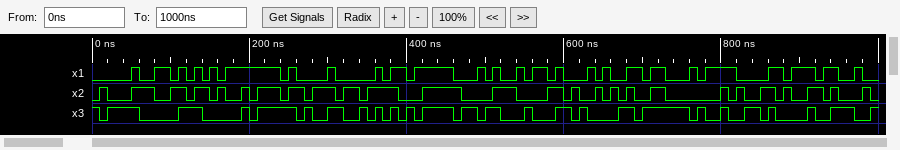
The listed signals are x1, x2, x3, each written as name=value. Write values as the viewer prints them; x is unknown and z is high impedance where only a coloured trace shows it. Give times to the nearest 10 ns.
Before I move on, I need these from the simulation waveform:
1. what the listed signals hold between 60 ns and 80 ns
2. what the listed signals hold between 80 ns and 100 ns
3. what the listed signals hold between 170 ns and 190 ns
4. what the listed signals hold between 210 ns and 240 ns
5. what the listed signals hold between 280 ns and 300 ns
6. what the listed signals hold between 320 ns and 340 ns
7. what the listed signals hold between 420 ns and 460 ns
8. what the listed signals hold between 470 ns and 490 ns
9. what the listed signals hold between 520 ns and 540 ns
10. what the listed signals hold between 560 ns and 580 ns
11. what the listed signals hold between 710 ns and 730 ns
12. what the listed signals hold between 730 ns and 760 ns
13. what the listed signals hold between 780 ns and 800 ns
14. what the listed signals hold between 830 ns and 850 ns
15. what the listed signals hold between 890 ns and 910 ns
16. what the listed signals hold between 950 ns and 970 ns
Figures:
x1=0, x2=1, x3=0
x1=1, x2=0, x3=0
x1=1, x2=0, x3=0
x1=1, x2=1, x3=1
x1=0, x2=1, x3=0
x1=0, x2=1, x3=0
x1=1, x2=1, x3=1
x1=0, x2=0, x3=1
x1=0, x2=1, x3=0
x1=1, x2=0, x3=0
x1=1, x2=1, x3=1
x1=0, x2=0, x3=1
x1=1, x2=0, x3=0
x1=0, x2=0, x3=1
x1=1, x2=0, x3=0
x1=0, x2=0, x3=1
